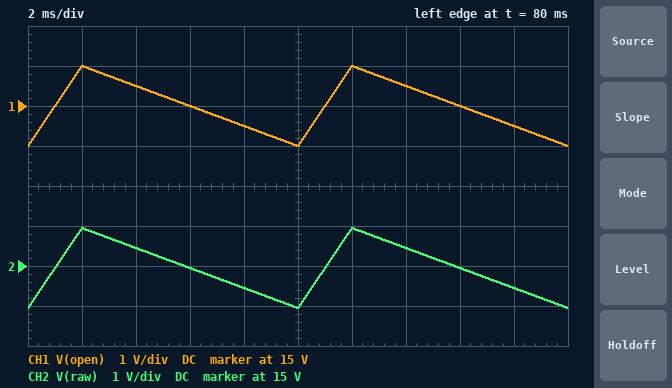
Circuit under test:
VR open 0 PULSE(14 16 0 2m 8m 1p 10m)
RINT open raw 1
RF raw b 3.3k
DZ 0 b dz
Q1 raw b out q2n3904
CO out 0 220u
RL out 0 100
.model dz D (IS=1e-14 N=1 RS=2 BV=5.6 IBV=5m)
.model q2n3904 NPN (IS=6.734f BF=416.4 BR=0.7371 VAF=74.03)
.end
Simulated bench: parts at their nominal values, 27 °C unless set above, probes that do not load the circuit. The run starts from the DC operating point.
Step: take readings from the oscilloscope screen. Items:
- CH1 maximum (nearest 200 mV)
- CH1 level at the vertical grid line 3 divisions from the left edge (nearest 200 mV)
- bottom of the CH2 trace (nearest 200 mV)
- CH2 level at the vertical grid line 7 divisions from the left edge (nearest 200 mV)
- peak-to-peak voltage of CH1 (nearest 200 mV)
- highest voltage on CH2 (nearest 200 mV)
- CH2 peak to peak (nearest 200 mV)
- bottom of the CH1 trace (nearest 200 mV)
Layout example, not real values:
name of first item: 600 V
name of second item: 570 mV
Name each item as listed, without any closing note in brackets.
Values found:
CH1 maximum: 16.0 V
CH1 level at the vertical grid line 3 divisions from the left edge: 15.0 V
bottom of the CH2 trace: 14.0 V
CH2 level at the vertical grid line 7 divisions from the left edge: 15.4 V
peak-to-peak voltage of CH1: 2.0 V
highest voltage on CH2: 16.0 V
CH2 peak to peak: 2.0 V
bottom of the CH1 trace: 14.0 V
